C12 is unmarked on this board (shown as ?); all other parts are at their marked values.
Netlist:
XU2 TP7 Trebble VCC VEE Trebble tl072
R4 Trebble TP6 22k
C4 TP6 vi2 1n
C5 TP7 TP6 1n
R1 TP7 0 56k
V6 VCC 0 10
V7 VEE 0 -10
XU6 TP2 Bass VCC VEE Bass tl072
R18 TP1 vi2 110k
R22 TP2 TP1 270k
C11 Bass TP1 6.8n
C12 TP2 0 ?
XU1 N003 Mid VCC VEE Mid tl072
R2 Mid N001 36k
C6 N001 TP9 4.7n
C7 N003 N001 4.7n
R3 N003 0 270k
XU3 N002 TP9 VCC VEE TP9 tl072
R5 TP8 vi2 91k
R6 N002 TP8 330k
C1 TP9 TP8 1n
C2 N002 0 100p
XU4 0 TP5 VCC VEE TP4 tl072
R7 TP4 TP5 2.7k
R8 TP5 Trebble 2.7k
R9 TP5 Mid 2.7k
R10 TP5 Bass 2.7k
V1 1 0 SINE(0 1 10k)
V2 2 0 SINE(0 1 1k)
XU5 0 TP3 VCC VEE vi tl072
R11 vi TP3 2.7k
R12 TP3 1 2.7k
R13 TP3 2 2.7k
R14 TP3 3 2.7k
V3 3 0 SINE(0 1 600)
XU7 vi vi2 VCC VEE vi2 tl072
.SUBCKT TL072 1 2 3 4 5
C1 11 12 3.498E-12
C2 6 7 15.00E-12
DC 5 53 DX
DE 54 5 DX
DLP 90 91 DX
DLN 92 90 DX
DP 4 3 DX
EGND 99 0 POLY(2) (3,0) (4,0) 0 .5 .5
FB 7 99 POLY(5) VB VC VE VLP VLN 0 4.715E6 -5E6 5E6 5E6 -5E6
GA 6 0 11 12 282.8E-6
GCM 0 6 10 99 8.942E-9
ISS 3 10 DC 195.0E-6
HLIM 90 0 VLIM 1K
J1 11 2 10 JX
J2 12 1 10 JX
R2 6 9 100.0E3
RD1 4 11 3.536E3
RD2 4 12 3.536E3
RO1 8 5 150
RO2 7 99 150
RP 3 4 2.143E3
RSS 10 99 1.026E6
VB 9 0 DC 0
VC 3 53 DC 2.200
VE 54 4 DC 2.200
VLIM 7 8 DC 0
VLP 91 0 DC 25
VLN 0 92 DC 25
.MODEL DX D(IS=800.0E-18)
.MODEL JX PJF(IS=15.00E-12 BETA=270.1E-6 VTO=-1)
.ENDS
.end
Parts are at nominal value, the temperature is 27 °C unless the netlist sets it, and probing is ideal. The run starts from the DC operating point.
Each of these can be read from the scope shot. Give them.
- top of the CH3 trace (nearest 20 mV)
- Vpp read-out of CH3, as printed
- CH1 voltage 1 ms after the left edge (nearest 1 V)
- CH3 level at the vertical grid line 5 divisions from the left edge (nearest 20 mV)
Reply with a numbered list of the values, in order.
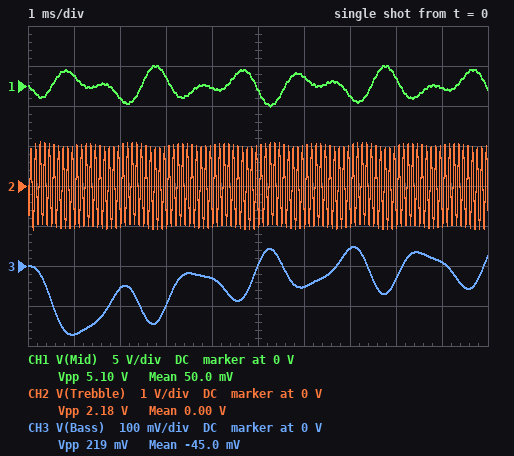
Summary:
1. 40 mV
2. 219 mV
3. 1 V
4. 0 V
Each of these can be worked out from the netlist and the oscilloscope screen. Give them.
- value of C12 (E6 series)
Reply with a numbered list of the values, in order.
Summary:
1. 6.8 nF
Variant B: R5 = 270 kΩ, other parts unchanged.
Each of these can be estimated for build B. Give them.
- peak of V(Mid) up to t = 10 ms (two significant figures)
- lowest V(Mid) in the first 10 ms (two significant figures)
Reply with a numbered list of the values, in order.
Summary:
1. 2.9 V
2. -2.9 V
